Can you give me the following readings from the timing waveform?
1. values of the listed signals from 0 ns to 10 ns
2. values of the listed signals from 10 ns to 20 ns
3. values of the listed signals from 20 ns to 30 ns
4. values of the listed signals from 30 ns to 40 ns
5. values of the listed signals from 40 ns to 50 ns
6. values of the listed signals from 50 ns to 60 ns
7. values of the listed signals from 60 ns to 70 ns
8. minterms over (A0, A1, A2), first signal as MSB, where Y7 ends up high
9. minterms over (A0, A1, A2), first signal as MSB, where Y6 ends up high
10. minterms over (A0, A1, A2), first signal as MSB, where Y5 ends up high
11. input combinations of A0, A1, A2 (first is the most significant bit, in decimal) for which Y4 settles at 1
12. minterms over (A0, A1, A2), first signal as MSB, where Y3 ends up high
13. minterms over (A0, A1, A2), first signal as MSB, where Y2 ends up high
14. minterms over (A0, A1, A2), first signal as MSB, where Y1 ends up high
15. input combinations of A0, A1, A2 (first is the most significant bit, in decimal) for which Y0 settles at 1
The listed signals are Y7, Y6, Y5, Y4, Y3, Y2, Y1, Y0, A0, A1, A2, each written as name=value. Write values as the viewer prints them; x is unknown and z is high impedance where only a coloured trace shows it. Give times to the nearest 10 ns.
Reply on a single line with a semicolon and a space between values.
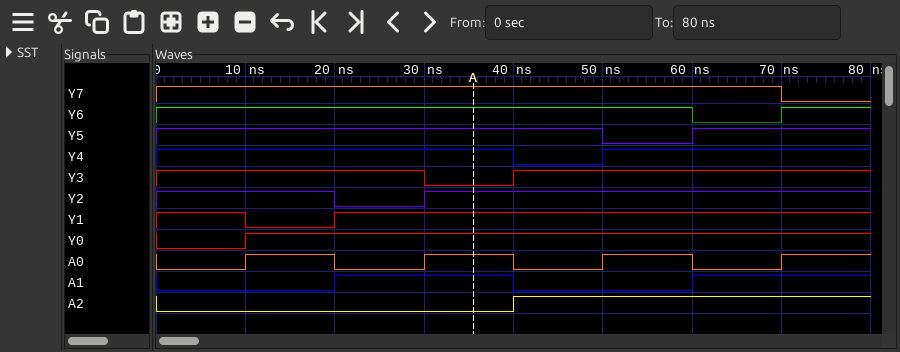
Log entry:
Y7=1, Y6=1, Y5=1, Y4=1, Y3=1, Y2=1, Y1=1, Y0=0, A0=0, A1=0, A2=0; Y7=1, Y6=1, Y5=1, Y4=1, Y3=1, Y2=1, Y1=0, Y0=1, A0=1, A1=0, A2=0; Y7=1, Y6=1, Y5=1, Y4=1, Y3=1, Y2=0, Y1=1, Y0=1, A0=0, A1=1, A2=0; Y7=1, Y6=1, Y5=1, Y4=1, Y3=0, Y2=1, Y1=1, Y0=1, A0=1, A1=1, A2=0; Y7=1, Y6=1, Y5=1, Y4=0, Y3=1, Y2=1, Y1=1, Y0=1, A0=0, A1=0, A2=1; Y7=1, Y6=1, Y5=0, Y4=1, Y3=1, Y2=1, Y1=1, Y0=1, A0=1, A1=0, A2=1; Y7=1, Y6=0, Y5=1, Y4=1, Y3=1, Y2=1, Y1=1, Y0=1, A0=0, A1=1, A2=1; 0, 1, 2, 3, 4, 5, 6; 0, 1, 2, 4, 5, 6, 7; 0, 1, 2, 3, 4, 6, 7; 0, 2, 3, 4, 5, 6, 7; 0, 1, 2, 3, 4, 5, 7; 0, 1, 3, 4, 5, 6, 7; 0, 1, 2, 3, 5, 6, 7; 1, 2, 3, 4, 5, 6, 7
